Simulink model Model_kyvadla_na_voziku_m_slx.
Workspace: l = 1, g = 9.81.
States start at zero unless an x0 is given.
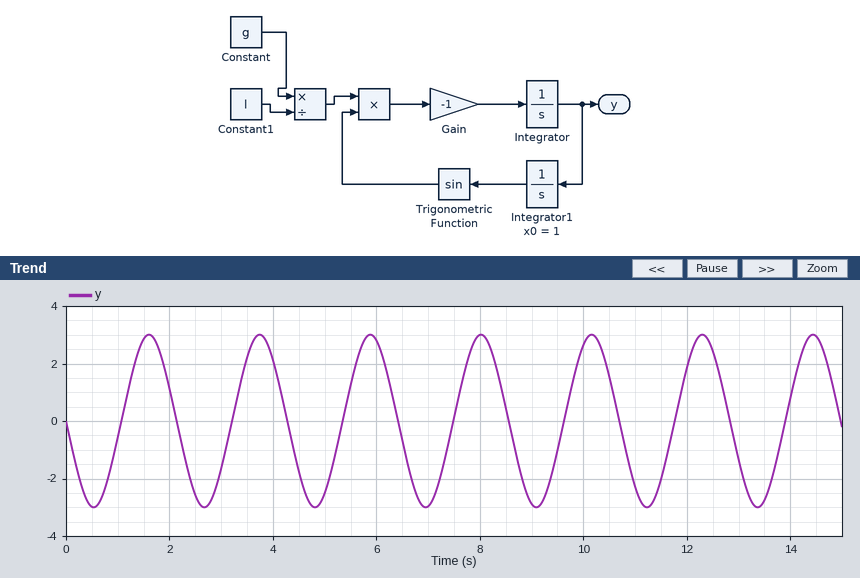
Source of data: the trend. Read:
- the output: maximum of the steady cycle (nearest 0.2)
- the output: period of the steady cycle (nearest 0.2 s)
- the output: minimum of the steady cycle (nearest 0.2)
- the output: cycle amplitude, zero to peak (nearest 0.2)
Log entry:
3.0
2.2 s
-3.0
3.0
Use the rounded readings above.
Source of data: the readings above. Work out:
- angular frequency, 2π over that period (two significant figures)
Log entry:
2.9 rad/s
